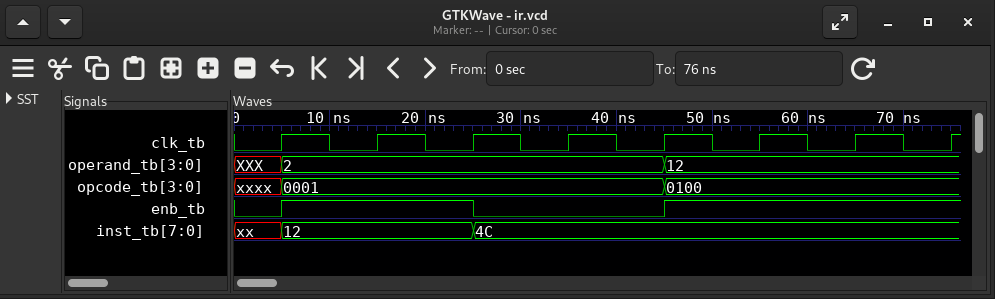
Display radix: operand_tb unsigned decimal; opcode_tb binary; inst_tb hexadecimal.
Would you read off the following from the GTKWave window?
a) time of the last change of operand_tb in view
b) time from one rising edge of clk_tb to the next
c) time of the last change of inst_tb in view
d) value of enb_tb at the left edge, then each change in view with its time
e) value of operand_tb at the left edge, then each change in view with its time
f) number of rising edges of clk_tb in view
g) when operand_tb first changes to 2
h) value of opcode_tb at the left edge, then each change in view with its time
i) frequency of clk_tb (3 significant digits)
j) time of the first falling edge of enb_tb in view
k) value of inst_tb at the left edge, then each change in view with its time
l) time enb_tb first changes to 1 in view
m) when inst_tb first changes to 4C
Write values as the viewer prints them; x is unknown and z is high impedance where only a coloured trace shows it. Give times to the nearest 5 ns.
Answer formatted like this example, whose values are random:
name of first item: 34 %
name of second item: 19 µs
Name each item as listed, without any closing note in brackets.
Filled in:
time of the last change of operand_tb in view: 45 ns
time from one rising edge of clk_tb to the next: 10 ns
time of the last change of inst_tb in view: 25 ns
value of enb_tb at the left edge, then each change in view with its time: 0, 1 at 5 ns, 0 at 25 ns, 1 at 45 ns
value of operand_tb at the left edge, then each change in view with its time: XXX, 2 at 5 ns, 12 at 45 ns
number of rising edges of clk_tb in view: 8
when operand_tb first changes to 2: 5 ns
value of opcode_tb at the left edge, then each change in view with its time: xxxx, 0001 at 5 ns, 0100 at 45 ns
frequency of clk_tb: 100 MHz
time of the first falling edge of enb_tb in view: 25 ns
value of inst_tb at the left edge, then each change in view with its time: xx, 12 at 5 ns, 4C at 25 ns
time enb_tb first changes to 1 in view: 5 ns
when inst_tb first changes to 4C: 25 ns
